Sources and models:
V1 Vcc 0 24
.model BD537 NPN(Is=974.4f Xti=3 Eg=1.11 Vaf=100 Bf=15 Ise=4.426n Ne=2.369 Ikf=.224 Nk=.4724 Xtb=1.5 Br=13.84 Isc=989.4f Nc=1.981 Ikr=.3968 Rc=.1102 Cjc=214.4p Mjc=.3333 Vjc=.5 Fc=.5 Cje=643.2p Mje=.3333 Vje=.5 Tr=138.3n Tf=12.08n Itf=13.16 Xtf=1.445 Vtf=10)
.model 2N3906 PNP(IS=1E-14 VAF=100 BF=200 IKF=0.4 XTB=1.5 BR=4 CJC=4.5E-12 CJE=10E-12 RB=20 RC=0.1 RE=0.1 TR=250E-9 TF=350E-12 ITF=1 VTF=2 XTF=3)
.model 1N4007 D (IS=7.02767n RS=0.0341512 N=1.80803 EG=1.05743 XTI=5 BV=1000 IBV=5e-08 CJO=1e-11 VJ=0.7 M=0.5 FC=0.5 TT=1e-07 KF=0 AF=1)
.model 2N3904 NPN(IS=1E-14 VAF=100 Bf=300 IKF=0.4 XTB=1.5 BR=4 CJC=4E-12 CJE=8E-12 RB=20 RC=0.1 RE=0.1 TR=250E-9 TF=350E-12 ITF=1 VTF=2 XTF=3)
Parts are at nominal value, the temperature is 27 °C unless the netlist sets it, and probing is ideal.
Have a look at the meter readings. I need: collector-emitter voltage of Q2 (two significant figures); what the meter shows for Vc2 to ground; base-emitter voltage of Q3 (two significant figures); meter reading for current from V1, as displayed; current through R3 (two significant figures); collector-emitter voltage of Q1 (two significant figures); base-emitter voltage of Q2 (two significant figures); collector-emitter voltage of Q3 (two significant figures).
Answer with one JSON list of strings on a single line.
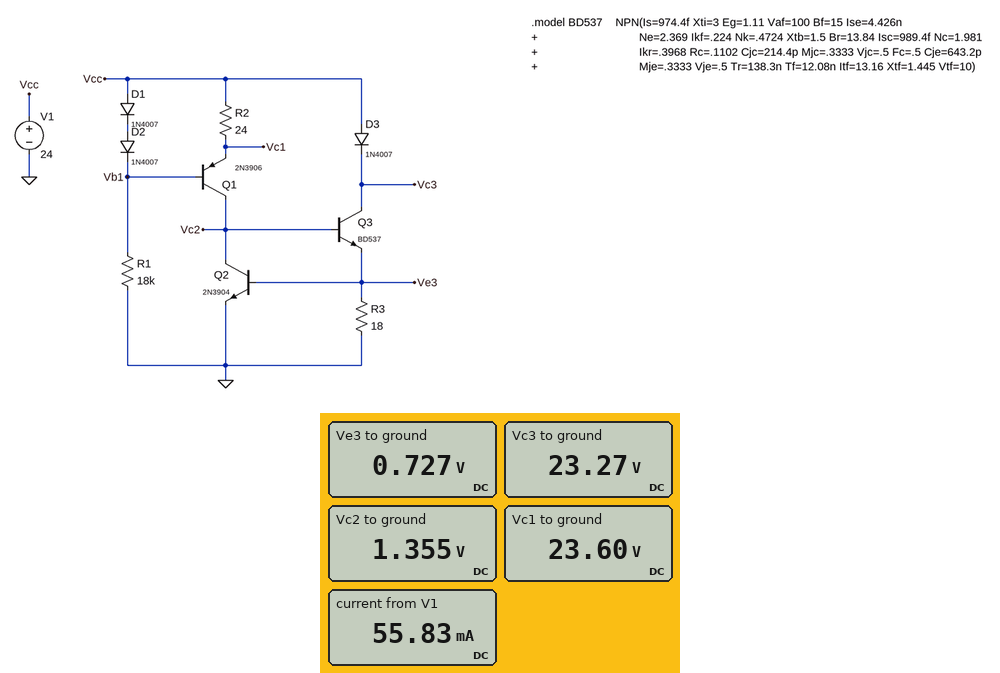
["1.4 V", "1.355 V", "630 mV", "55.83 mA", "40 mA", "-22 V", "730 mV", "23 V"]
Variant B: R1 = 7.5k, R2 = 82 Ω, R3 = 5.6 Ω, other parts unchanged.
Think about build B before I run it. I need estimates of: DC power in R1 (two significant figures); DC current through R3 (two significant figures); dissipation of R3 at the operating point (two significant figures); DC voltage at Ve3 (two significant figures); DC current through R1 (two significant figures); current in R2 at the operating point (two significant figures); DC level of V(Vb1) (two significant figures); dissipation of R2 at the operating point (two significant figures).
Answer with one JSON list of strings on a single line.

["69 mW", "92 mA", "48 mW", "520 mV", "3.0 mA", "6.3 mA", "23 V", "3.2 mW"]
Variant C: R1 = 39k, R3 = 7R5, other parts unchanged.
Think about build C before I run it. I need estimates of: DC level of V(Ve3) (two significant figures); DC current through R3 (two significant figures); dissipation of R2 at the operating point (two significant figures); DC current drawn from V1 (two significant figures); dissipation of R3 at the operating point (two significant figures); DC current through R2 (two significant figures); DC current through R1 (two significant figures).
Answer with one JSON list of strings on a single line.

["710 mV", "94 mA", "4.5 mW", "100 mA", "67 mW", "14 mA", "590 µA"]
